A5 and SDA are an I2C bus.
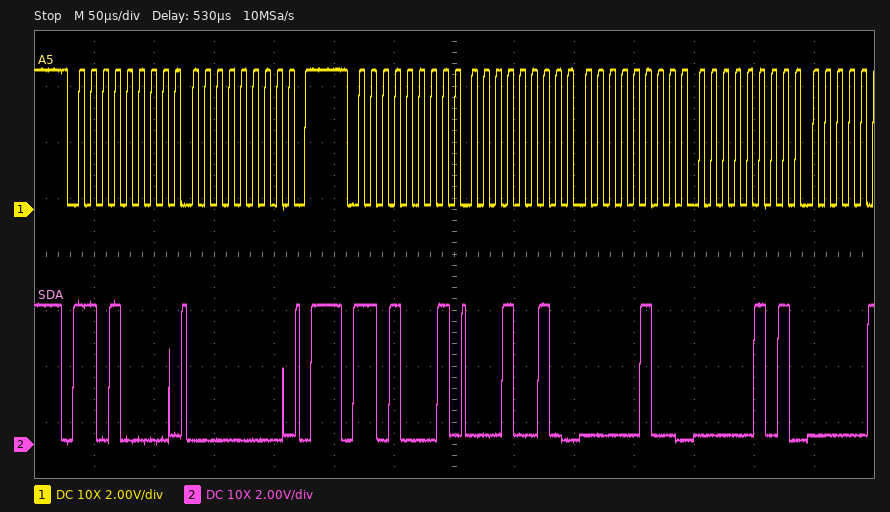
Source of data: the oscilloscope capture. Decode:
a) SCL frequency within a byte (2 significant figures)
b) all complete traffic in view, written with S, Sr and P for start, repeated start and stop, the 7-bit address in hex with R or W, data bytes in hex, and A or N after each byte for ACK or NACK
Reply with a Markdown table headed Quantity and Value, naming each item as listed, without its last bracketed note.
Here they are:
| Quantity | Value |
|---|---|
| SCL frequency within a byte | 100 kHz |
| all complete traffic in view, written with S, Sr and P for start, repeated start and stop, the 7-bit address in hex with R or W, data bytes in hex, and A or N after each byte for ACK or NACK | S 68W A 00 A P S 68R A 12 A 04 A 05 A |
